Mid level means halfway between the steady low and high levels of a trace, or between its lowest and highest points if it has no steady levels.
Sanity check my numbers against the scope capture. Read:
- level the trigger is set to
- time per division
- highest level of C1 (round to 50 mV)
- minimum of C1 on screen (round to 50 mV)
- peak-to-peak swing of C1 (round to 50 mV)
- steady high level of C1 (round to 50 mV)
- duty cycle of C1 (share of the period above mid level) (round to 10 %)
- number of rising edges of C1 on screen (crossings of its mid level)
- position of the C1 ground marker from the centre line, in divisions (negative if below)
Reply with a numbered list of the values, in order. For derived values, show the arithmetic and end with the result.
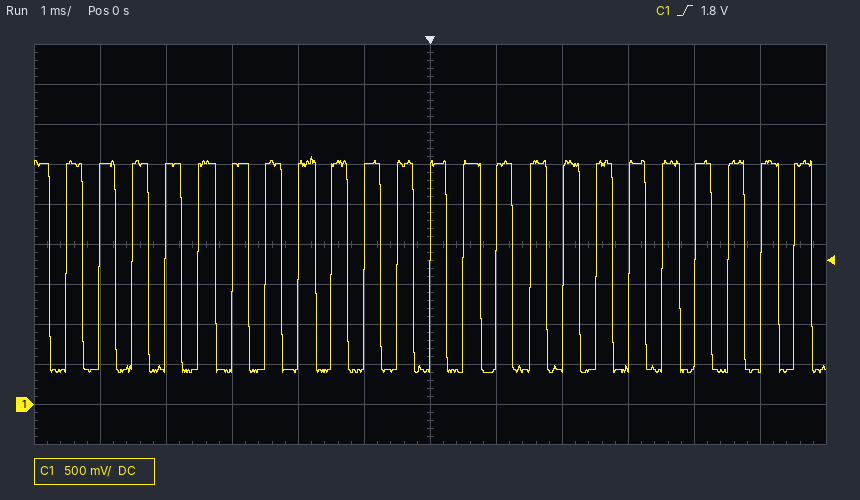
1. 1.8 V
2. 1 ms
3. 3.10 V
4. 400 mV
5. 3.10 V − (400 mV) = 2.70 V
6. 3.00 V
7. 50 %
8. 23
9. -4.0 div
